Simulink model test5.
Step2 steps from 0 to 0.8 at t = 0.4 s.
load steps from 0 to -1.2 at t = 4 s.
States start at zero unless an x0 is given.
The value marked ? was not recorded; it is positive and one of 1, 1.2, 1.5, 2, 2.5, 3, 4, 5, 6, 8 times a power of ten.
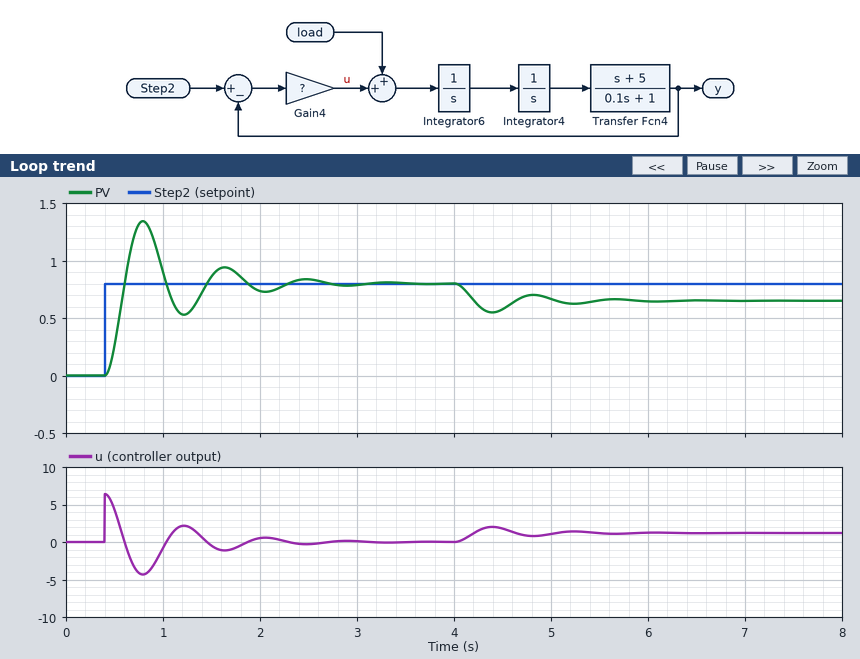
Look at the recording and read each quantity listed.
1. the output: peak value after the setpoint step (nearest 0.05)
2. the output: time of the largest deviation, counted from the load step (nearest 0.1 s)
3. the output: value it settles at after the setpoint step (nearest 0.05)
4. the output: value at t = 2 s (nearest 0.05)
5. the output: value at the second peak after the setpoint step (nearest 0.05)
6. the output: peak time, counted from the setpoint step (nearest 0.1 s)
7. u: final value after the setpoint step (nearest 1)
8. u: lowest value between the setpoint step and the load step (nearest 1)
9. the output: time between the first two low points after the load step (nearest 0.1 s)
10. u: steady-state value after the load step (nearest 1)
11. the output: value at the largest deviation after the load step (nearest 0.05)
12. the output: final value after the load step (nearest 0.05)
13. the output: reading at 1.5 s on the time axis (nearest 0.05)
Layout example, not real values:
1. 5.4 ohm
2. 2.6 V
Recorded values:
1. 1.35
2. 0.4 s
3. 0.80
4. 0.75
5. 0.95
6. 0.4 s
7. 0
8. -4
9. 0.8 s
10. 1
11. 0.55
12. 0.65
13. 0.85
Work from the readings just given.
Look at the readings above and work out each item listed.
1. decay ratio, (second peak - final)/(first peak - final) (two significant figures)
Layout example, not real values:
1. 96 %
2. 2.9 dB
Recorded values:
1. 0.27
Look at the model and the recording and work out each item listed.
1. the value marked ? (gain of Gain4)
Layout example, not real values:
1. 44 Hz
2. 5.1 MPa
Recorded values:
1. 8
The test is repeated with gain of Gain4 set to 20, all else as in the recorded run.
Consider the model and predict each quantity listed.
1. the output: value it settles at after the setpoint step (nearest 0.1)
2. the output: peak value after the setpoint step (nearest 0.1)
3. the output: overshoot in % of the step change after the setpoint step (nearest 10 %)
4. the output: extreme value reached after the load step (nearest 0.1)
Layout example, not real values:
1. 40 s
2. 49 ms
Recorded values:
1. 0.8
2. 1.4
3. 70 %
4. 0.7
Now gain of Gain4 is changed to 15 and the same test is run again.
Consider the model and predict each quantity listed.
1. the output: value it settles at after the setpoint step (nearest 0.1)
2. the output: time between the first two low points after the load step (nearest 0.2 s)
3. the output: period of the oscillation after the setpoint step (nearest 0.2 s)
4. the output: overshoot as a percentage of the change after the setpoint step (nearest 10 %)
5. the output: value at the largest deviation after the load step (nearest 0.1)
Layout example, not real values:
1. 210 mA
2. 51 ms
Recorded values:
1. 0.8
2. 0.6 s
3. 0.6 s
4. 70 %
5. 0.7
